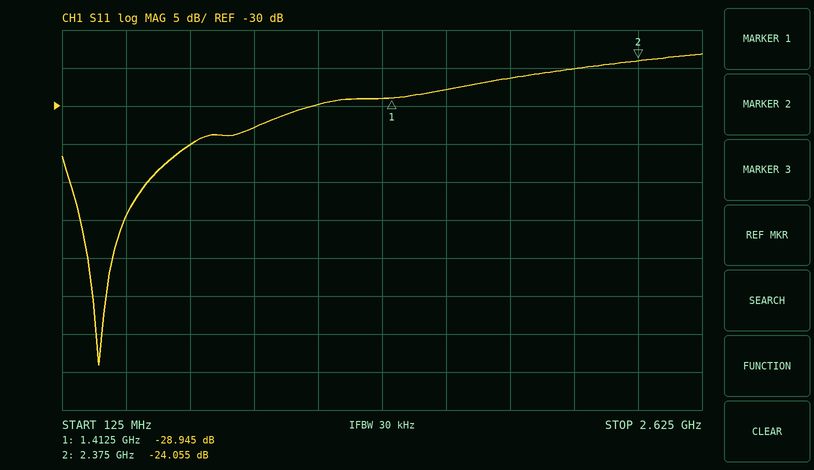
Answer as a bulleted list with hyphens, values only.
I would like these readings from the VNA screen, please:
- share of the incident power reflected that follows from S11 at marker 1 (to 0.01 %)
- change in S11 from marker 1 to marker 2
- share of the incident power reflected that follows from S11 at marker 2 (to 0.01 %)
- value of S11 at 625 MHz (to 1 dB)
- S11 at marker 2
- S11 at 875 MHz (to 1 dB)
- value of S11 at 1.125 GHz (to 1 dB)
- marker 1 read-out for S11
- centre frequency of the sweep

- 0.13 %
- 4.890 dB
- 0.39 %
- -35 dB
- -24.055 dB
- -33 dB
- -30 dB
- -28.945 dB
- 1.375 GHz
